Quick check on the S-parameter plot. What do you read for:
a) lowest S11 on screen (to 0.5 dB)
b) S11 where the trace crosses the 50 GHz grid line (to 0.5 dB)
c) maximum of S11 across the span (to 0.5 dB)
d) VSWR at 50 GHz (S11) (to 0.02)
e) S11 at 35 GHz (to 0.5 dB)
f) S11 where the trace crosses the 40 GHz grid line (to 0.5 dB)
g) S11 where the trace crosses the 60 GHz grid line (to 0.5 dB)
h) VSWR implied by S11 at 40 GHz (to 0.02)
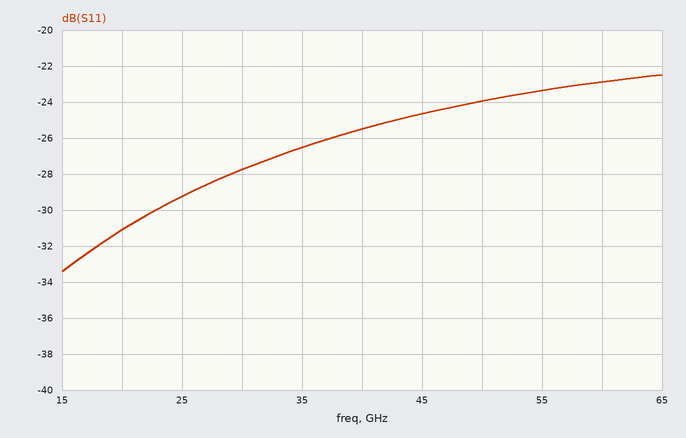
-33.5 dB
-24.0 dB
-22.5 dB
1.14
-26.5 dB
-25.5 dB
-23.0 dB
1.12
